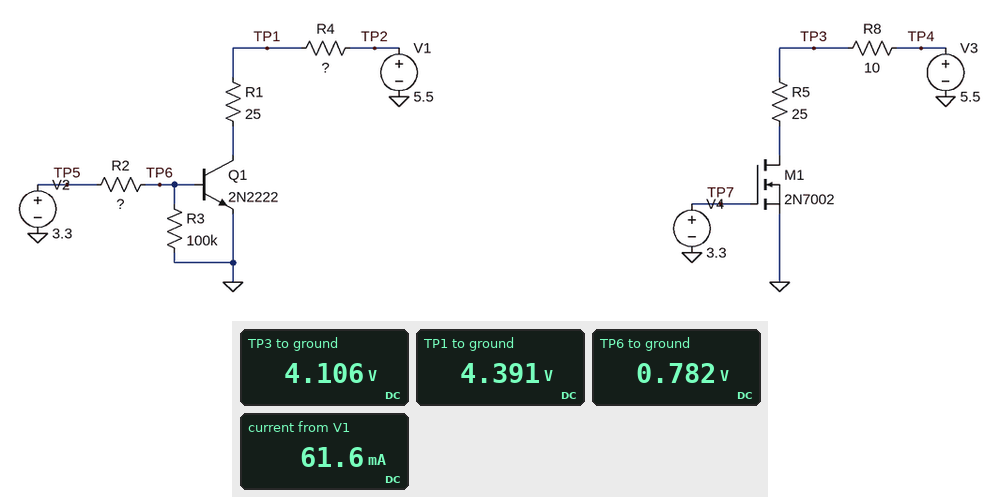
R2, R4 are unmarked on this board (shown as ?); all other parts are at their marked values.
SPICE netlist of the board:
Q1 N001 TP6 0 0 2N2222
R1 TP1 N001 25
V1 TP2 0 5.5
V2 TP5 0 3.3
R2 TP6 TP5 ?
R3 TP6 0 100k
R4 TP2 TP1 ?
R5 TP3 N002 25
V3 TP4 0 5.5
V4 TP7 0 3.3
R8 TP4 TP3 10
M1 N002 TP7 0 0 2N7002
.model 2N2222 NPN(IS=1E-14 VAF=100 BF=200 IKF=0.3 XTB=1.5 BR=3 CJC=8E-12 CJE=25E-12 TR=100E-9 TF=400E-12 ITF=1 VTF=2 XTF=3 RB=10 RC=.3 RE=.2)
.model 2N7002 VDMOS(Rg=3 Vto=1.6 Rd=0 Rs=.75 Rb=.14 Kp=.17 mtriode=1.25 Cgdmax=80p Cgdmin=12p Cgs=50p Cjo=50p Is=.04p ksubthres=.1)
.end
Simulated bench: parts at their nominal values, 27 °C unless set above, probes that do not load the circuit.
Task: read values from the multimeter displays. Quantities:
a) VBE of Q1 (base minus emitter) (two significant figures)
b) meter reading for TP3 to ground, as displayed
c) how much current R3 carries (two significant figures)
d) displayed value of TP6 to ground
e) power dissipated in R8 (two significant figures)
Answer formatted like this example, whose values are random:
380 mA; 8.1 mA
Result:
780 mV; 4.106 V; 7.8 µA; 0.782 V; 190 mW
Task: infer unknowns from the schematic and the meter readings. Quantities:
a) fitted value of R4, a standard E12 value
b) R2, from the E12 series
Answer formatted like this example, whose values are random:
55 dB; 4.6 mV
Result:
18 Ω; 6.8 kΩ
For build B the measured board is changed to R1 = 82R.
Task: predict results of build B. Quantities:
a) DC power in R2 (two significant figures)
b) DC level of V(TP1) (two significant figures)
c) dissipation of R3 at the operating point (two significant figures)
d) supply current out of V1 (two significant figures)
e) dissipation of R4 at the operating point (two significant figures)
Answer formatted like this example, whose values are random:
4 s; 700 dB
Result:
940 µW; 4.5 V; 6.0 µW; 53 mA; 51 mW
